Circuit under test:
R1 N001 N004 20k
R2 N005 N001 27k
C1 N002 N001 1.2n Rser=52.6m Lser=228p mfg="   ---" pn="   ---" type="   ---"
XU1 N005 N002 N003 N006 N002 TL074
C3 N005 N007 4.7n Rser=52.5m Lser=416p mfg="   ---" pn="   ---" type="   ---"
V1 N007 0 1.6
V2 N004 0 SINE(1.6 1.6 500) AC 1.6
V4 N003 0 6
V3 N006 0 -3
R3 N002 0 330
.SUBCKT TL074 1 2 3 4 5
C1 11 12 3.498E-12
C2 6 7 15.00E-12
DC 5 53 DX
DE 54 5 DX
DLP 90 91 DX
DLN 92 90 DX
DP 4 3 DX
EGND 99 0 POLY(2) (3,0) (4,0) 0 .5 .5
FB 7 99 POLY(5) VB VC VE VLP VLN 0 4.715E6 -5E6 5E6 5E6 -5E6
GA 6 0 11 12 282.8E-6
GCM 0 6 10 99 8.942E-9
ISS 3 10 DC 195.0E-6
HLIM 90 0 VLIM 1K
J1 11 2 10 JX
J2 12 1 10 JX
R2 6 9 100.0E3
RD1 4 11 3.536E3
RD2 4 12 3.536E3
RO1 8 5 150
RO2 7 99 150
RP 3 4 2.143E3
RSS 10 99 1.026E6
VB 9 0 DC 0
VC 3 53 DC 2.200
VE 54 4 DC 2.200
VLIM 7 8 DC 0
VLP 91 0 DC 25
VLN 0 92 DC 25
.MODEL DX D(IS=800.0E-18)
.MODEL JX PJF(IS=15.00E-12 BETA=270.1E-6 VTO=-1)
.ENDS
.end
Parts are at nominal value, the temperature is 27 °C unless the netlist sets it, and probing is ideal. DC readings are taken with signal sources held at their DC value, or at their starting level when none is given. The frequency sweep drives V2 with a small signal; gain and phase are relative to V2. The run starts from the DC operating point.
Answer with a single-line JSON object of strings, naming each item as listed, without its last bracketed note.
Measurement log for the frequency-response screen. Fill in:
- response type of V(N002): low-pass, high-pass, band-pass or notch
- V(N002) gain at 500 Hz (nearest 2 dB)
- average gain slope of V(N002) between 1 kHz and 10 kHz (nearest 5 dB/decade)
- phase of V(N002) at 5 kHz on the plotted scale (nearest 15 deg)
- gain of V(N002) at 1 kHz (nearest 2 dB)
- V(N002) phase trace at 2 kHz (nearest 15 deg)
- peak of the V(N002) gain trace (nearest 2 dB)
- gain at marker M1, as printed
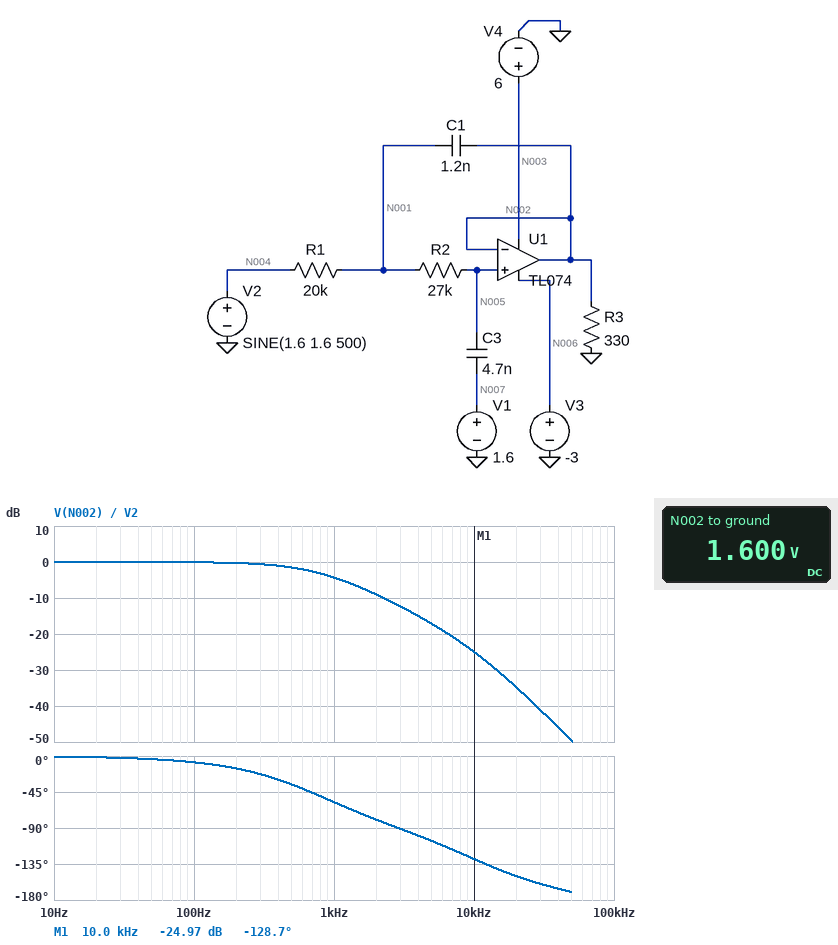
{"response type of V(N002): low-pass, high-pass, band-pass or notch": "low-pass", "V(N002) gain at 500 Hz": "-2 dB", "average gain slope of V(N002) between 1 kHz and 10 kHz": "-20 dB/decade", "phase of V(N002) at 5 kHz on the plotted scale": "-105 deg", "gain of V(N002) at 1 kHz": "-4 dB", "V(N002) phase trace at 2 kHz": "-75 deg", "peak of the V(N002) gain trace": "0 dB", "gain at marker M1, as printed": "-24.97 dB"}
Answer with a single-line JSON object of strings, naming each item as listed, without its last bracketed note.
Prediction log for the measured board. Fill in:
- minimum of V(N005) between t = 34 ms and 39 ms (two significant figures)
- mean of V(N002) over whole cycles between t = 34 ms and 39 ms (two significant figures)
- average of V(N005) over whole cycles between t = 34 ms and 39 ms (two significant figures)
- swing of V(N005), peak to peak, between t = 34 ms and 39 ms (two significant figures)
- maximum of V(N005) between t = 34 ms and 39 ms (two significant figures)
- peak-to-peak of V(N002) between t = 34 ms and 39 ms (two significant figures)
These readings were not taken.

{"minimum of V(N005) between t = 34 ms and 39 ms": "260 mV", "mean of V(N002) over whole cycles between t = 34 ms and 39 ms": "1.6 V", "average of V(N005) over whole cycles between t = 34 ms and 39 ms": "1.6 V", "swing of V(N005), peak to peak, between t = 34 ms and 39 ms": "2.7 V", "maximum of V(N005) between t = 34 ms and 39 ms": "2.9 V", "peak-to-peak of V(N002) between t = 34 ms and 39 ms": "2.7 V"}
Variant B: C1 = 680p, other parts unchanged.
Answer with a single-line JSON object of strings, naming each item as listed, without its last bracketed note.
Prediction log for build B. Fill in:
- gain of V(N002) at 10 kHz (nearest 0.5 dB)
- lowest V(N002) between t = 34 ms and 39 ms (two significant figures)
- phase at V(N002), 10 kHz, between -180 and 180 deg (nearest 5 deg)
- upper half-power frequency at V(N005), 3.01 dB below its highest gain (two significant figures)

{"gain of V(N002) at 10 kHz": "-23.5 dB", "lowest V(N002) between t = 34 ms and 39 ms": "270 mV", "phase at V(N002), 10 kHz, between -180 and 180 deg": "-115 deg", "upper half-power frequency at V(N005), 3.01 dB below its highest gain": "750 Hz"}
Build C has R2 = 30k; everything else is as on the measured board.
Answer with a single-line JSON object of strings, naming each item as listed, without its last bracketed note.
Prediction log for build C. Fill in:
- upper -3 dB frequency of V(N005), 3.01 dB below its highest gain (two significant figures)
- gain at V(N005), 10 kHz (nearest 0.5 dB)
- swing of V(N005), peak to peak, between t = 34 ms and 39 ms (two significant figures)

{"upper -3 dB frequency of V(N005), 3.01 dB below its highest gain": "720 Hz", "gain at V(N005), 10 kHz": "-25.5 dB", "swing of V(N005), peak to peak, between t = 34 ms and 39 ms": "2.6 V"}
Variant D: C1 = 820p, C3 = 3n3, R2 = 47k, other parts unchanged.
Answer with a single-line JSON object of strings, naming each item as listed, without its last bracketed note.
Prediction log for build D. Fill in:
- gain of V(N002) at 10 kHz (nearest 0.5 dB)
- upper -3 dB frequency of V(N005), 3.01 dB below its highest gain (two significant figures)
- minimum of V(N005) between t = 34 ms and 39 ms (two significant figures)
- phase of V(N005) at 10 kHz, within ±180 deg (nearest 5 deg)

{"gain of V(N002) at 10 kHz": "-24.5 dB", "upper -3 dB frequency of V(N005), 3.01 dB below its highest gain": "760 Hz", "minimum of V(N005) between t = 34 ms and 39 ms": "260 mV", "phase of V(N005) at 10 kHz, within ±180 deg": "-125 deg"}
